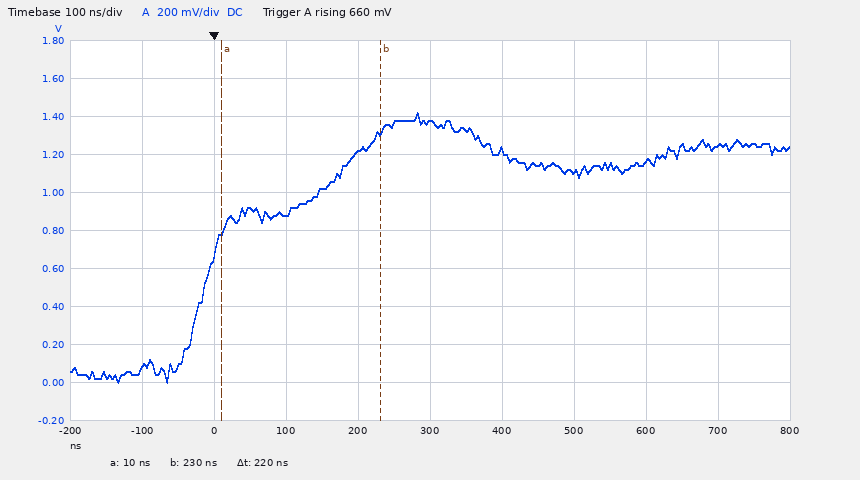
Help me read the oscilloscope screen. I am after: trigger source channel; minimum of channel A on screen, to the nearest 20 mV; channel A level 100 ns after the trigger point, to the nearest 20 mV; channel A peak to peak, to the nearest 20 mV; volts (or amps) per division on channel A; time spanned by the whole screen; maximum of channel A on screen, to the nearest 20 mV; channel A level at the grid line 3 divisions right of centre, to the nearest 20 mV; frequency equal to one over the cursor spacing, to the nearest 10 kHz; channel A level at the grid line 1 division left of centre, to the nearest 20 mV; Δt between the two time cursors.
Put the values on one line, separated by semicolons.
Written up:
channel A; 0 mV; 880 mV; 1.42 V; 200 mV; 1 µs; 1.42 V; 1.16 V; 4.55 MHz; 1.22 V; 220 ns
